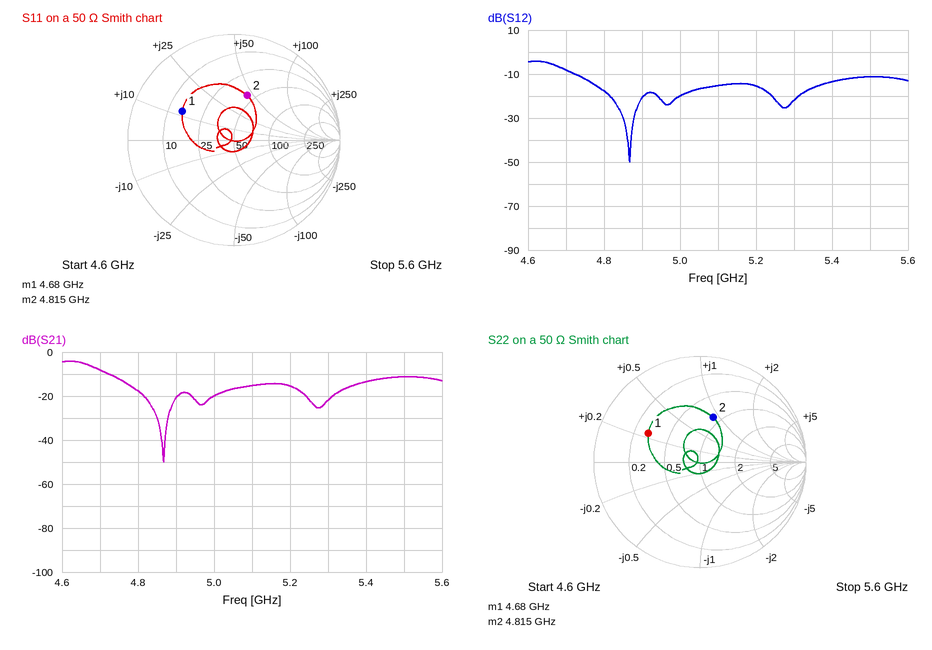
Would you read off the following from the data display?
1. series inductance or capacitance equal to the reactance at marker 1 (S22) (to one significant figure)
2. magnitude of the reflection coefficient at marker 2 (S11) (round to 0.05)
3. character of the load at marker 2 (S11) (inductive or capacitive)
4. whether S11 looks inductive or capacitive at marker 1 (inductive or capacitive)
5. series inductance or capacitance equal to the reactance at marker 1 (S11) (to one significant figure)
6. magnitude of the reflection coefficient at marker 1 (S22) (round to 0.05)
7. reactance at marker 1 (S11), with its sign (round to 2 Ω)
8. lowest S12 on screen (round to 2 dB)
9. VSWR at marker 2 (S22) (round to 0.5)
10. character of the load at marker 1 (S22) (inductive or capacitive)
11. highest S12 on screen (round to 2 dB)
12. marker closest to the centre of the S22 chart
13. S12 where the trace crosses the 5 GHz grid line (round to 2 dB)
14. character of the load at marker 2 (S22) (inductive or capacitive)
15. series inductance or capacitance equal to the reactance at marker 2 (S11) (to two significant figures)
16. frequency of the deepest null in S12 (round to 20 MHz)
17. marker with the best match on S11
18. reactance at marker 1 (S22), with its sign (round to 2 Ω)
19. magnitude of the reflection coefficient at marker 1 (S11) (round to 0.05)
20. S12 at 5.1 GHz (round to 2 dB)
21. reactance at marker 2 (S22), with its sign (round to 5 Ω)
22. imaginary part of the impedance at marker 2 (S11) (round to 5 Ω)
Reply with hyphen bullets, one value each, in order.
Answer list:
- 400 pH
- 0.45
- inductive
- inductive
- 400 pH
- 0.55
- +12 Ω
- -50 dB
- 2.5
- inductive
- -4 dB
- marker 2
- -20 dB
- inductive
- 1.5 nH
- 4.86 GHz
- marker 2
- +12 Ω
- 0.55
- -16 dB
- +45 Ω
- +45 Ω
